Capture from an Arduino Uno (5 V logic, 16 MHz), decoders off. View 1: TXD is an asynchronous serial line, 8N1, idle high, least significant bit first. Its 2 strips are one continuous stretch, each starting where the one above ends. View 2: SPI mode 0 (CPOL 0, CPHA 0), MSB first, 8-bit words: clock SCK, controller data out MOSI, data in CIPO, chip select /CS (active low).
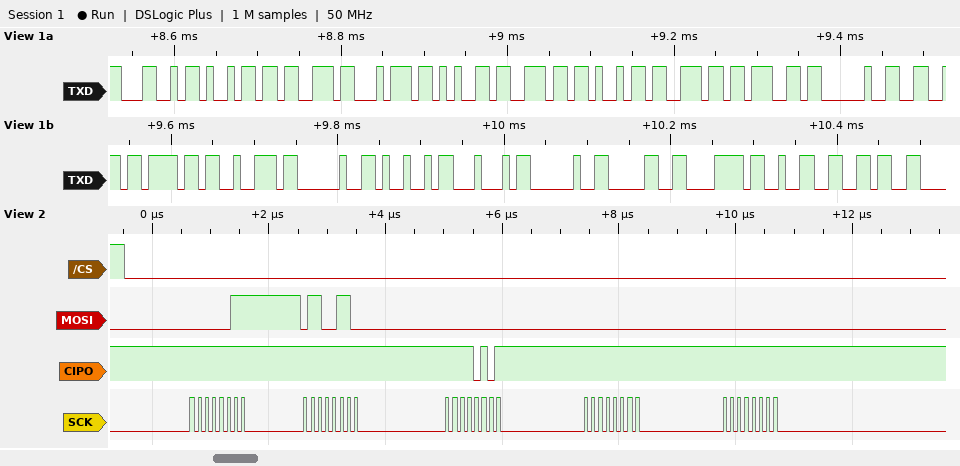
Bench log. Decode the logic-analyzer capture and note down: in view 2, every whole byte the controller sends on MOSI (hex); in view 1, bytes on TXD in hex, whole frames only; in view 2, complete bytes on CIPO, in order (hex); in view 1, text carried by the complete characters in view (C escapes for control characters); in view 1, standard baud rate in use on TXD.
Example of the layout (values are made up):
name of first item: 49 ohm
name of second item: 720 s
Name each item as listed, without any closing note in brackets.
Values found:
in view 2, every whole byte the controller sends on MOSI: 03 66 00 00 00
in view 1, bytes on TXD in hex, whole frames only: 4C 69 73 74 65 6E 69 6E 67 20 66 6F 72 20 49 44 20 30 78 32 36
in view 2, complete bytes on CIPO, in order: FF FF F5 FF FF
in view 1, text carried by the complete characters in view: "Listening for ID 0x26"
in view 1, standard baud rate in use on TXD: 115200 baud
